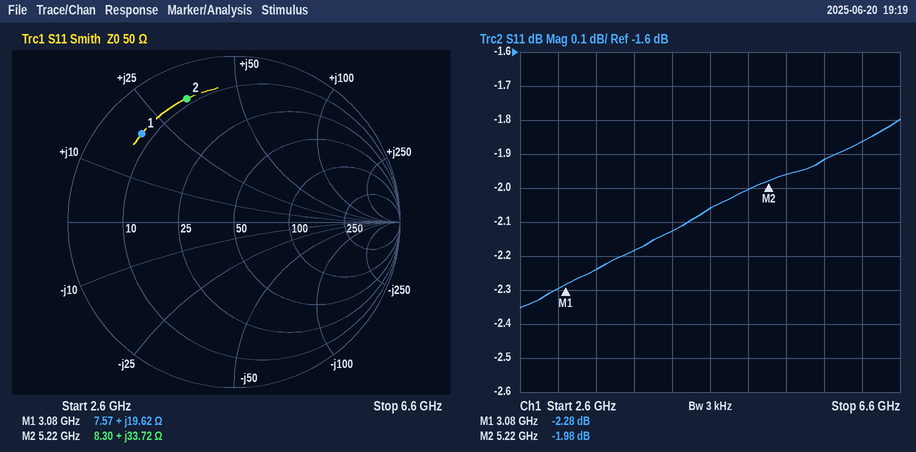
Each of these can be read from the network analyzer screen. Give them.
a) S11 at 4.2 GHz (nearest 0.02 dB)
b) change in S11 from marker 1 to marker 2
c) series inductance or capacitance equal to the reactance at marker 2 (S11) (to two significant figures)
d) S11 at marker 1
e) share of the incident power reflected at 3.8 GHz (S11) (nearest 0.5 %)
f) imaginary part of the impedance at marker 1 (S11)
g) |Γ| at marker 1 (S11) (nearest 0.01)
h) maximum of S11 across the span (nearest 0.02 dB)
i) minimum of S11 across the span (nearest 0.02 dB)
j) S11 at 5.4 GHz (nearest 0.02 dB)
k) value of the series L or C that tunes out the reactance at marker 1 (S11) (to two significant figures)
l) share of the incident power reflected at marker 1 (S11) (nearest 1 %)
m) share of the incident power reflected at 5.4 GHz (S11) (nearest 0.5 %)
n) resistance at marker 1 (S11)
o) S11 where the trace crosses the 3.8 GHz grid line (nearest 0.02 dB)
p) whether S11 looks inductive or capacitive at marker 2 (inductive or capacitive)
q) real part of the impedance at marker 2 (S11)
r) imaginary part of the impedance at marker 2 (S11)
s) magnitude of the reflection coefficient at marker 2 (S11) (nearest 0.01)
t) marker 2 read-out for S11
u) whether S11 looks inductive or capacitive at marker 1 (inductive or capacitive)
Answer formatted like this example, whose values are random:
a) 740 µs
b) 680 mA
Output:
a) -2.12 dB
b) 0.30 dB
c) 1.0 nH
d) -2.28 dB
e) 60.5 %
f) +19.62 Ω
g) 0.77
h) -1.80 dB
i) -2.36 dB
j) -1.96 dB
k) 2.6 pF
l) 59 %
m) 63.5 %
n) 7.57 Ω
o) -2.18 dB
p) inductive
q) 8.30 Ω
r) +33.72 Ω
s) 0.80
t) -1.98 dB
u) inductive
